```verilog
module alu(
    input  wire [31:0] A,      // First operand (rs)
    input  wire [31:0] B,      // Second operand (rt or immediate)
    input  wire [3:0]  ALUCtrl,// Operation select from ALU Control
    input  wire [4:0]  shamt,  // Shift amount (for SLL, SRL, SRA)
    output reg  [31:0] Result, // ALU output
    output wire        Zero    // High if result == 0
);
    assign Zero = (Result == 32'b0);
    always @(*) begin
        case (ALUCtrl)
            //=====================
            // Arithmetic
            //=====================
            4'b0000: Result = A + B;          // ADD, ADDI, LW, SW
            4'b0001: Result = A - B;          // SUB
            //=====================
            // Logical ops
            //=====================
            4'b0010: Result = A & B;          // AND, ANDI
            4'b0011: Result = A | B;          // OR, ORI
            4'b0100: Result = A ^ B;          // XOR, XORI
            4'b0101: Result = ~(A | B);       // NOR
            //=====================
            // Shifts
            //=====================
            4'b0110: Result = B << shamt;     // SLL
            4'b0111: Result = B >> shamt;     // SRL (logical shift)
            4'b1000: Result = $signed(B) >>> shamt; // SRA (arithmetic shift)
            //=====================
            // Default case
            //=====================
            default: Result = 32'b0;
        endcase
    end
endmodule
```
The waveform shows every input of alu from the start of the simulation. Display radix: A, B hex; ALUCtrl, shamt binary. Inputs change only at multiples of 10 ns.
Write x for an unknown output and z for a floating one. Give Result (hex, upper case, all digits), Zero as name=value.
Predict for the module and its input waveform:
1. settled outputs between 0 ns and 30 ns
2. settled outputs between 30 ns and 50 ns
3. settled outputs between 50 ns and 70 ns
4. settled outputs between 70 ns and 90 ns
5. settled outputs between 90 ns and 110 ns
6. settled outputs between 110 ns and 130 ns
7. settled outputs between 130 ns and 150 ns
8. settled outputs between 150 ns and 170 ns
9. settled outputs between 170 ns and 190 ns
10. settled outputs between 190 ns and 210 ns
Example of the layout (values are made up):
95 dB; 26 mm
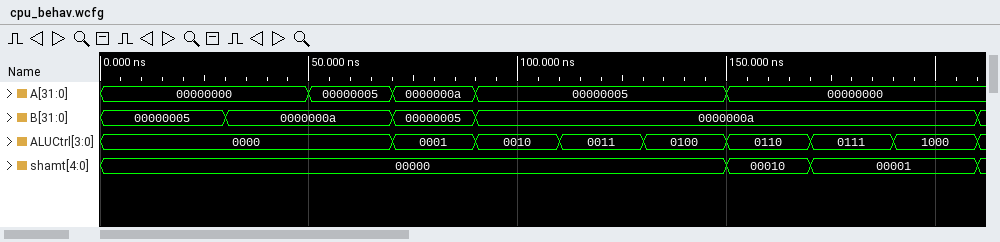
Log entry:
Result=00000005, Zero=0; Result=0000000A, Zero=0; Result=0000000F, Zero=0; Result=00000005, Zero=0; Result=00000000, Zero=1; Result=0000000F, Zero=0; Result=0000000F, Zero=0; Result=00000028, Zero=0; Result=00000005, Zero=0; Result=00000005, Zero=0
